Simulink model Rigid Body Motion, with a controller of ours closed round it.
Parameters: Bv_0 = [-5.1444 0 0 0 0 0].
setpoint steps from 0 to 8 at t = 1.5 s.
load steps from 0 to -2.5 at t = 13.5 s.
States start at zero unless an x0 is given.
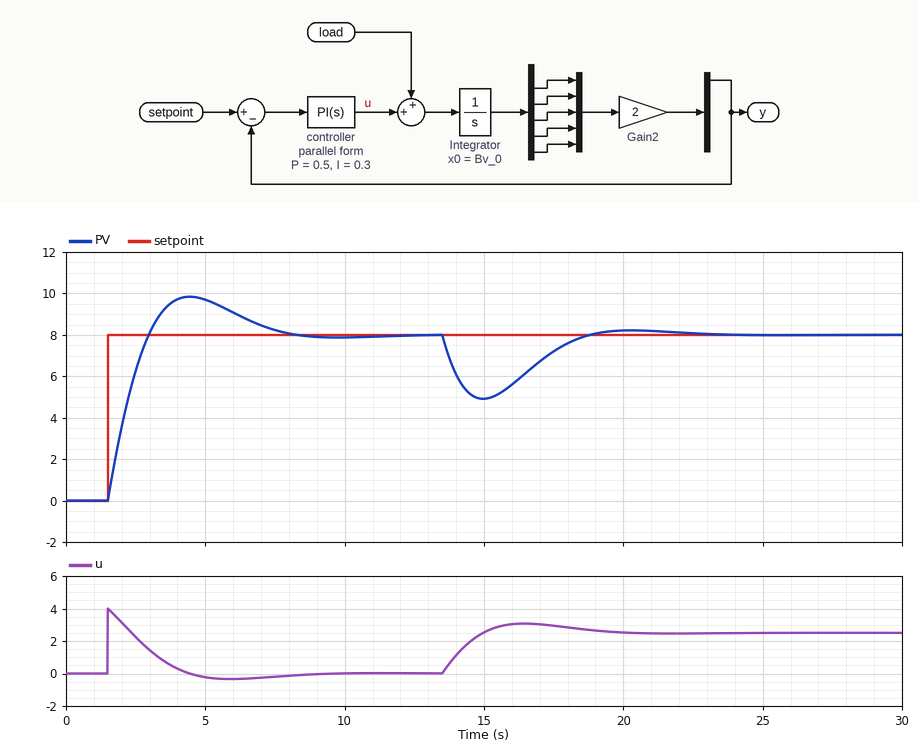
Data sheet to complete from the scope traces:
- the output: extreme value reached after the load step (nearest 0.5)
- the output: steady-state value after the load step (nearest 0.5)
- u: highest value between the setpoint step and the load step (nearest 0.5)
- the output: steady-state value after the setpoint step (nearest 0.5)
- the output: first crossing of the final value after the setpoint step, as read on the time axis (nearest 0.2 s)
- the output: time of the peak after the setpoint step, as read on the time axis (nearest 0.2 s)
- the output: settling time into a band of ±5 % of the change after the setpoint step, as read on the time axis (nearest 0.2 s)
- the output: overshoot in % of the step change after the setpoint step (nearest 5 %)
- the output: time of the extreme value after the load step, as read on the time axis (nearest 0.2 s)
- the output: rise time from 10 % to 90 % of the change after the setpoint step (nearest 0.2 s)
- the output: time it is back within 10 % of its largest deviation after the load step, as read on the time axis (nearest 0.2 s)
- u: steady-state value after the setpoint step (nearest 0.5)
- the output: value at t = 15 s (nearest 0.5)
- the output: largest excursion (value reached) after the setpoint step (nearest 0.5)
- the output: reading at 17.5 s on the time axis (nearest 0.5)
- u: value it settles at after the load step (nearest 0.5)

5.0
8.0
4.0
8.0
3.0 s
4.4 s
7.2 s
25 %
15.0 s
1.2 s
18.2 s
0.0
5.0
10.0
7.0
2.5
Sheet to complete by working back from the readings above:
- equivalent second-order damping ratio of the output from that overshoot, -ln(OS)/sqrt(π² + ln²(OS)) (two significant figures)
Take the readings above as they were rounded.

0.40
